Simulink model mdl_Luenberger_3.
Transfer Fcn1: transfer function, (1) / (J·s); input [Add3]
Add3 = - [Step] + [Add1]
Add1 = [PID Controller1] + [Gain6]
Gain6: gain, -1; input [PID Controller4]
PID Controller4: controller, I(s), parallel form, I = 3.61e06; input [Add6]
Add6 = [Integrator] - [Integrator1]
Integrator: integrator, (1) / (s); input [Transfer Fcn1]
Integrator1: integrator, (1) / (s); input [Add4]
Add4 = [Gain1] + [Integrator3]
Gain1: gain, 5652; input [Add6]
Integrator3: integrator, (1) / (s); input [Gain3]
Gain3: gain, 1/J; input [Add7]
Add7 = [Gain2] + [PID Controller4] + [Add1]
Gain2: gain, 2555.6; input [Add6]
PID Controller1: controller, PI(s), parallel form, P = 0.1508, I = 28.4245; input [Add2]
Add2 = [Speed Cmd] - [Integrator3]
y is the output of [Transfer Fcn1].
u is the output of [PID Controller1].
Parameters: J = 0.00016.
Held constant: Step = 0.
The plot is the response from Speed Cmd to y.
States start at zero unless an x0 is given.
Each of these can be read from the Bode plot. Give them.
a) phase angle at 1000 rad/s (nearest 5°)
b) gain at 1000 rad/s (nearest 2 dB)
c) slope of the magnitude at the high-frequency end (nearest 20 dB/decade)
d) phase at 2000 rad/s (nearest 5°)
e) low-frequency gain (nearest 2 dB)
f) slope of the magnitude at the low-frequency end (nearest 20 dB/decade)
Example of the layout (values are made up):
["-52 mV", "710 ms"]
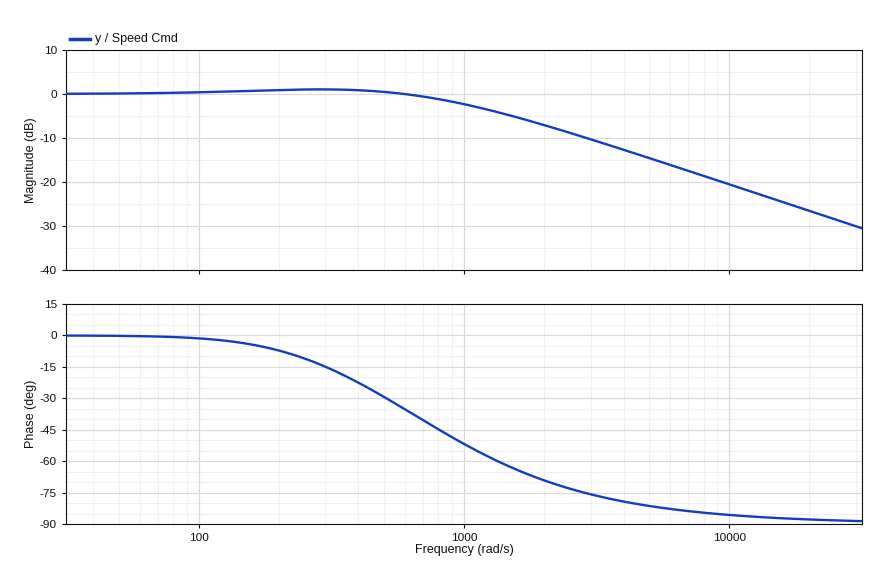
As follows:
["-50°", "-2 dB", "-20 dB/decade", "-70°", "0 dB", "0 dB/decade"]
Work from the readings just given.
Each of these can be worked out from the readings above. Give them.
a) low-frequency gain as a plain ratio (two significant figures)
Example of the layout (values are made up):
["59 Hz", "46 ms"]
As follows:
["1.0"]
